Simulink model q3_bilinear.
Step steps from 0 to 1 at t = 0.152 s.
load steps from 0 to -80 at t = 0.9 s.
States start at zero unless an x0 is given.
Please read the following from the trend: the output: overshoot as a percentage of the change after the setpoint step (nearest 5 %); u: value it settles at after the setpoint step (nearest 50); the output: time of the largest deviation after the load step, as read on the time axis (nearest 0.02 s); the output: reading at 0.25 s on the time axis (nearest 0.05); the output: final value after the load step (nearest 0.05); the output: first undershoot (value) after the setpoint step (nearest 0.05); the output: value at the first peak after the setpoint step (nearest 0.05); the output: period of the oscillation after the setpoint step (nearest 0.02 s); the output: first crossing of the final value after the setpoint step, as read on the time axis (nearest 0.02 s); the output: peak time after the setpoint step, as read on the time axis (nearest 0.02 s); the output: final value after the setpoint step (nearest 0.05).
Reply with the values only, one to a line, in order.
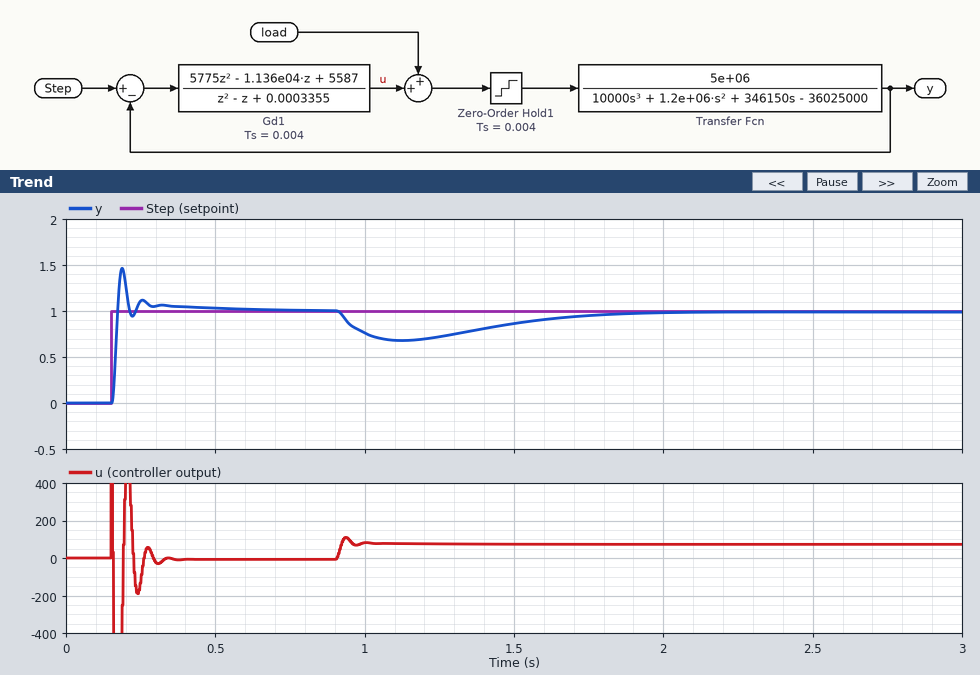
45 %
0
1.12 s
1.10
1.00
0.95
1.45
0.06 s
0.18 s
0.18 s
1.00
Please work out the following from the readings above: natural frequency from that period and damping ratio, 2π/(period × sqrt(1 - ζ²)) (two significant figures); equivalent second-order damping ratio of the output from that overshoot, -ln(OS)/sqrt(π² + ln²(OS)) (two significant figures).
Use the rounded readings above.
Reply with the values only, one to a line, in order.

110 rad/s
0.25
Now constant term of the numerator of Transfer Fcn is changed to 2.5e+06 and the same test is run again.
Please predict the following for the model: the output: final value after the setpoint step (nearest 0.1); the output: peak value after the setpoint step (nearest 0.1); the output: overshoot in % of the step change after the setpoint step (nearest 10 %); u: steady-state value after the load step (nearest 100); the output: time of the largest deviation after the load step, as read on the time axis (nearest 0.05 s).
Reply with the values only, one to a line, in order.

1.0
1.3
30 %
100
1.15 s
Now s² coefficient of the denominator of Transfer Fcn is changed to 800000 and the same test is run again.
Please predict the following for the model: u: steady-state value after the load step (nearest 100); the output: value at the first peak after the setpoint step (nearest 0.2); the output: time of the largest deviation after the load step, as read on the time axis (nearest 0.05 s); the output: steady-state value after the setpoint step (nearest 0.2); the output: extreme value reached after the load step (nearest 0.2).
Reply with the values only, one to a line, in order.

100
1.8
1.15 s
1.0
0.6
